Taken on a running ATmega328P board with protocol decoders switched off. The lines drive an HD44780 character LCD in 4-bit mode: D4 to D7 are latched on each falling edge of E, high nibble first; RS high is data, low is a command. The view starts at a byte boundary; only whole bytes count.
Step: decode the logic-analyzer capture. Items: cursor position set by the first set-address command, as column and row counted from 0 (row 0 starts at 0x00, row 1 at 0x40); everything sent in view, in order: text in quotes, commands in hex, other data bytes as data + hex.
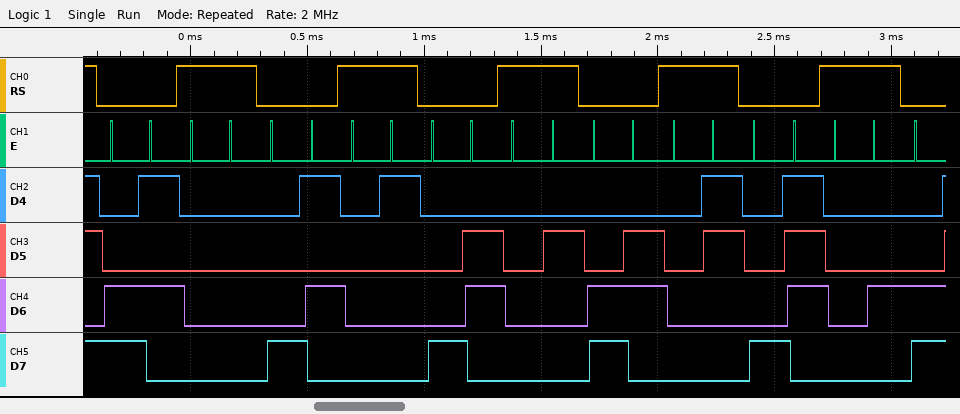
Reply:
column 5, row 1
0xC5 data 00 0x85 data 01 0x86 data 02 0xC6 data 03 0x87 data 04
